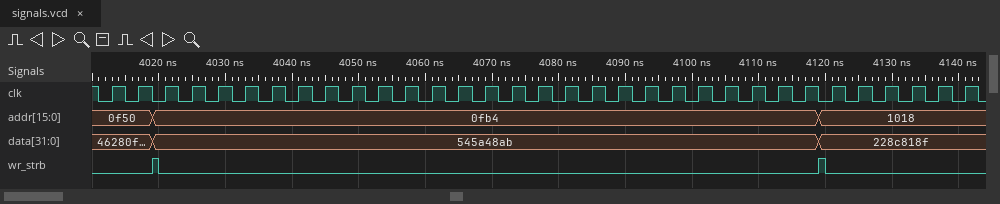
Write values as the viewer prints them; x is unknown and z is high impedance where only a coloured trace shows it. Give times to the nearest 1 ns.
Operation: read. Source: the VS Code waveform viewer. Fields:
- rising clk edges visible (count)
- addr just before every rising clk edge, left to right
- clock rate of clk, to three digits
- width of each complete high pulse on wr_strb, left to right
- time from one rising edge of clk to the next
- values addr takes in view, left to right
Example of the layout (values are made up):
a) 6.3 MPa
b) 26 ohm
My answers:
a) 33
b) 0f50, 0f50, 0fb4, 0fb4, 0fb4, 0fb4, 0fb4, 0fb4, 0fb4, 0fb4, 0fb4, 0fb4, 0fb4, 0fb4, 0fb4, 0fb4, 0fb4, 0fb4, 0fb4, 0fb4, 0fb4, 0fb4, 0fb4, 0fb4, 0fb4, 0fb4, 0fb4, 1018, 1018, 1018, 1018, 1018, 1018
c) 250 MHz
d) 1 ns, 1 ns
e) 4 ns
f) 0f50, 0fb4, 1018
